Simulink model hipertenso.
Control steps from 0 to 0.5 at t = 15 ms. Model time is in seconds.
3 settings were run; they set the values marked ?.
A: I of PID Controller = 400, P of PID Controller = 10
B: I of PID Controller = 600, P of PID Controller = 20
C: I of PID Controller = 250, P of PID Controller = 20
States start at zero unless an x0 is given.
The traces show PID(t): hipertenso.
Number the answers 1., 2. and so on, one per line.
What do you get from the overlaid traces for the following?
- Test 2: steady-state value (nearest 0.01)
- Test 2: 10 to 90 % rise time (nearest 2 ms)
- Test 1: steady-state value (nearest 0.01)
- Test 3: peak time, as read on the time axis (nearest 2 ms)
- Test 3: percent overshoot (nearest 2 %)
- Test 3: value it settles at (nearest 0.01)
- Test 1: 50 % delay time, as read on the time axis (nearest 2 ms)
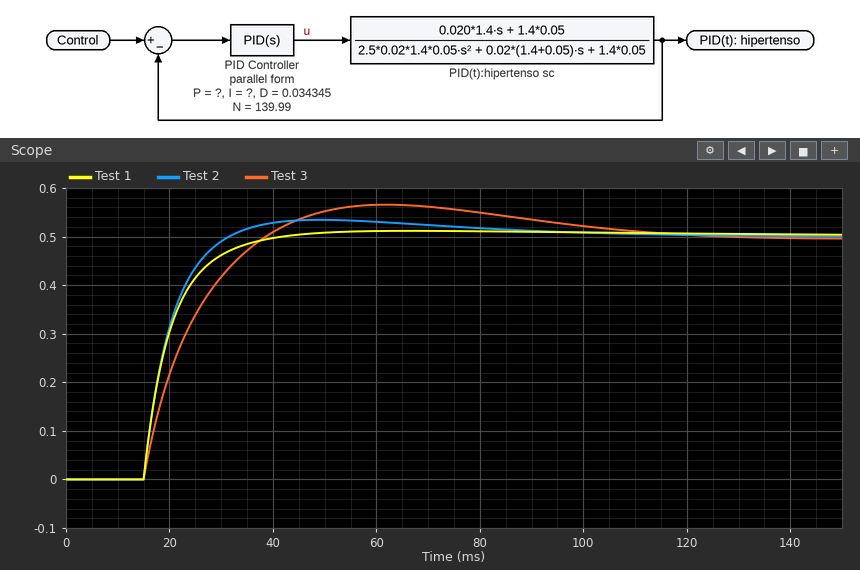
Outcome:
1. 0.50
2. 10 ms
3. 0.50
4. 62 ms
5. 14 %
6. 0.50
7. 18 ms
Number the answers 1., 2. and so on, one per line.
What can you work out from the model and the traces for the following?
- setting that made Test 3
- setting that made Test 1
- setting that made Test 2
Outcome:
1. A
2. C
3. B
